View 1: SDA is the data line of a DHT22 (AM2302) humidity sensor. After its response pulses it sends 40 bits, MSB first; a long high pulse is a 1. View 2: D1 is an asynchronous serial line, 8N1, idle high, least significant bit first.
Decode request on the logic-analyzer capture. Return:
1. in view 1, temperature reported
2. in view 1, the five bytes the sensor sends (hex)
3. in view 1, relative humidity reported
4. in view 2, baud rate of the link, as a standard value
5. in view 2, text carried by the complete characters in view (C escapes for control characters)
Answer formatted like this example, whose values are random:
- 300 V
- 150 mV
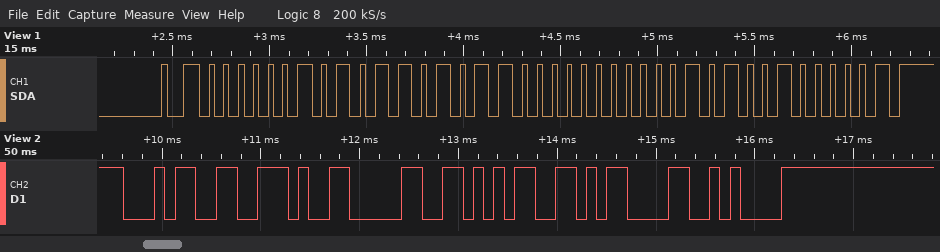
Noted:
- -1.0 °C
- 02 B5 80 0A 41
- 69.3 %
- 9600 baud
- "4.05\r\n"
